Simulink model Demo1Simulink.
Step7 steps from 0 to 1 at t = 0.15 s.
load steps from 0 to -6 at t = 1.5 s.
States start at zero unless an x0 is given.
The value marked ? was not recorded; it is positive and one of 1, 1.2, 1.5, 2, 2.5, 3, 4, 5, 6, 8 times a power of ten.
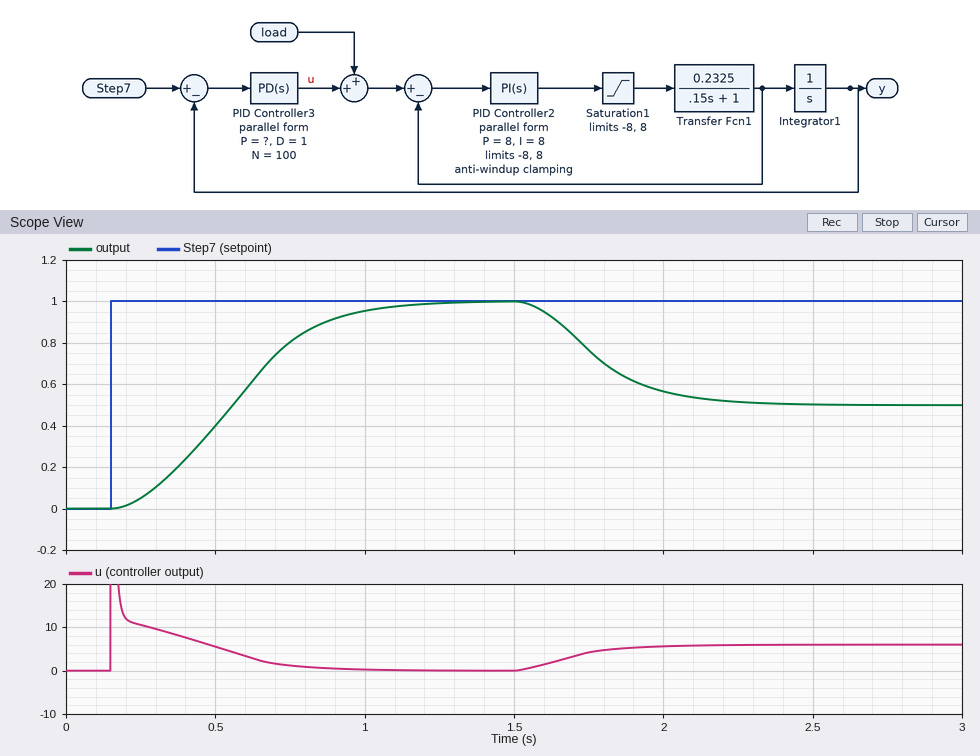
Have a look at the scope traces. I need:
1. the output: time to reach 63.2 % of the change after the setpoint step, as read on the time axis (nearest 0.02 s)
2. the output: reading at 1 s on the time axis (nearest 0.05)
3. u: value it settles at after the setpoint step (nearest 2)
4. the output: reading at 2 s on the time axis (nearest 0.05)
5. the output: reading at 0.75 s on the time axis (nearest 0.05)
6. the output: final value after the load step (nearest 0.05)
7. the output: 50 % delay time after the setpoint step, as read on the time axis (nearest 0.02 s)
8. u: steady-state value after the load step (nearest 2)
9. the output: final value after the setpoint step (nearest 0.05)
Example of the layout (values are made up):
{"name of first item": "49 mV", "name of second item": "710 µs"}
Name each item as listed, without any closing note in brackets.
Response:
{"the output: time to reach 63.2 % of the change after the setpoint step, as read on the time axis": "0.64 s", "the output: reading at 1 s on the time axis": "0.95", "u: value it settles at after the setpoint step": "0", "the output: reading at 2 s on the time axis": "0.55", "the output: reading at 0.75 s on the time axis": "0.80", "the output: final value after the load step": "0.50", "the output: 50 % delay time after the setpoint step, as read on the time axis": "0.56 s", "u: steady-state value after the load step": "6", "the output: final value after the setpoint step": "1.00"}
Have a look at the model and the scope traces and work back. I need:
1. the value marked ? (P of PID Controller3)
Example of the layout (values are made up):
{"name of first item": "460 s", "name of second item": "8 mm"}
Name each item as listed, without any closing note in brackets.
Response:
{"the value marked ?": "12"}
